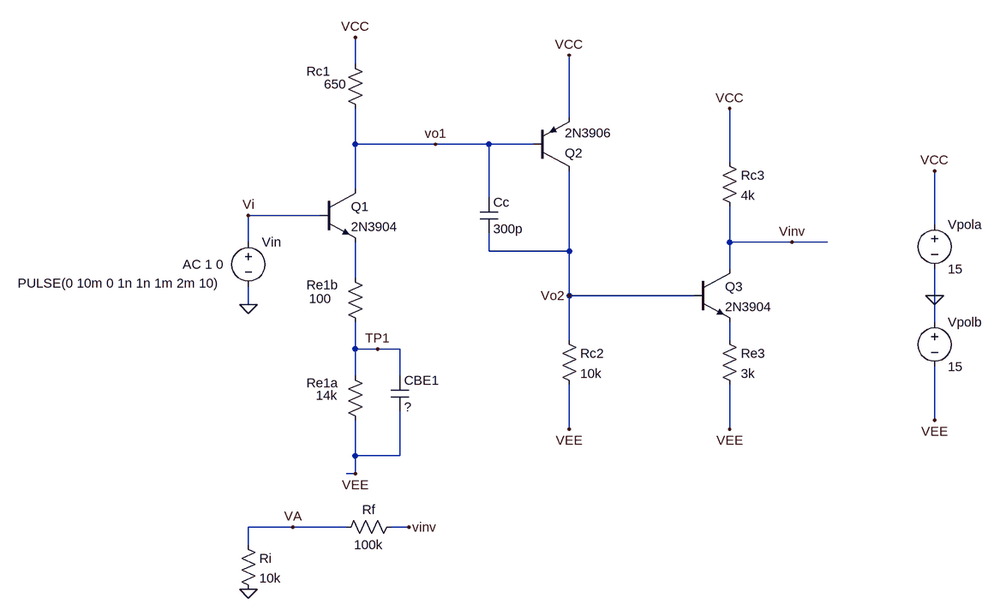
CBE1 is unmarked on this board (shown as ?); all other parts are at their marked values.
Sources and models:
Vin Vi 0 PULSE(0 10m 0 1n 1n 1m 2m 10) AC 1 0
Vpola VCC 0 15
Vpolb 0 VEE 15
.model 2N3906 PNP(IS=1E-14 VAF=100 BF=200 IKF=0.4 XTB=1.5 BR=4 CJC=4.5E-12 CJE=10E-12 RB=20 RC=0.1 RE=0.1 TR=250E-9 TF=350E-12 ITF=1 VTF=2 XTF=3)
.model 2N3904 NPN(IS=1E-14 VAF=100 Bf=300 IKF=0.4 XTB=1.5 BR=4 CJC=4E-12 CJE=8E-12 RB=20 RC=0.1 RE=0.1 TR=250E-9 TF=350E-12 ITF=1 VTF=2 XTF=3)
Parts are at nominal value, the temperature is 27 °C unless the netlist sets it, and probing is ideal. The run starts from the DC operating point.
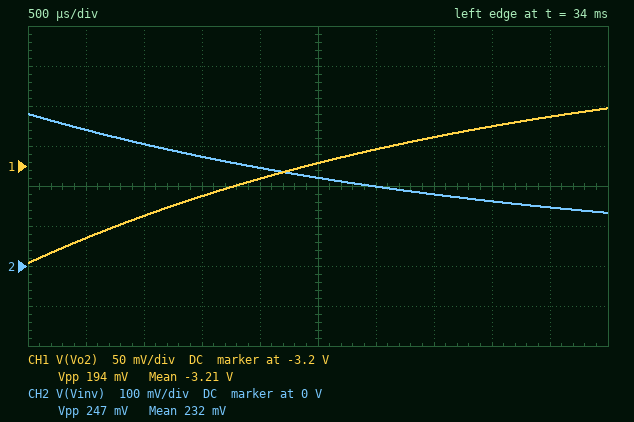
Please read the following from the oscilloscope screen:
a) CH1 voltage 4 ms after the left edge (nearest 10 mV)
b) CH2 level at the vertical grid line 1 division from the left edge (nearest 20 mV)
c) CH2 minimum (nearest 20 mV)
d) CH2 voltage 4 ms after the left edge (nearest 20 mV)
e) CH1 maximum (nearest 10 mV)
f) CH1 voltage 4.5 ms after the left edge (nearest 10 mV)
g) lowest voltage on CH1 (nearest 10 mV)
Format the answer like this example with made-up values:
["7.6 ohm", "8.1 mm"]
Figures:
["-3.15 V", "340 mV", "140 mV", "160 mV", "-3.13 V", "-3.14 V", "-3.32 V"]
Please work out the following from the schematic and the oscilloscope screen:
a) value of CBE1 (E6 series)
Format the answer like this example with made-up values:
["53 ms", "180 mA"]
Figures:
["33 µF"]
